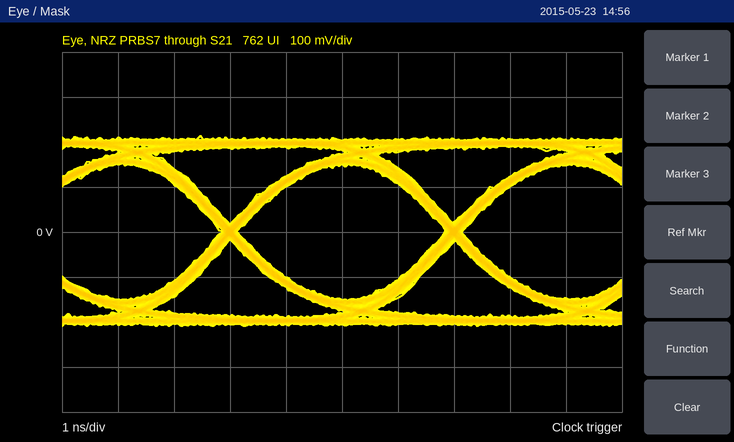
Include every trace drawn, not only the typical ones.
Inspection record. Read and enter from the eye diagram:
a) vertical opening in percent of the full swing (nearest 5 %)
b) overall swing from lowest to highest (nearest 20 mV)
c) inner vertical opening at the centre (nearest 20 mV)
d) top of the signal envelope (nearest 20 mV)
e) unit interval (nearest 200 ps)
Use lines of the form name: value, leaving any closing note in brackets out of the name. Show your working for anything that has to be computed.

vertical opening in percent of the full swing: 300 mV / 420 mV ≈ 71.4 %, so 70 % to the nearest 5 %
overall swing from lowest to highest: 420 mV
inner vertical opening at the centre: 300 mV
top of the signal envelope: 220 mV
unit interval: 4.0 ns
